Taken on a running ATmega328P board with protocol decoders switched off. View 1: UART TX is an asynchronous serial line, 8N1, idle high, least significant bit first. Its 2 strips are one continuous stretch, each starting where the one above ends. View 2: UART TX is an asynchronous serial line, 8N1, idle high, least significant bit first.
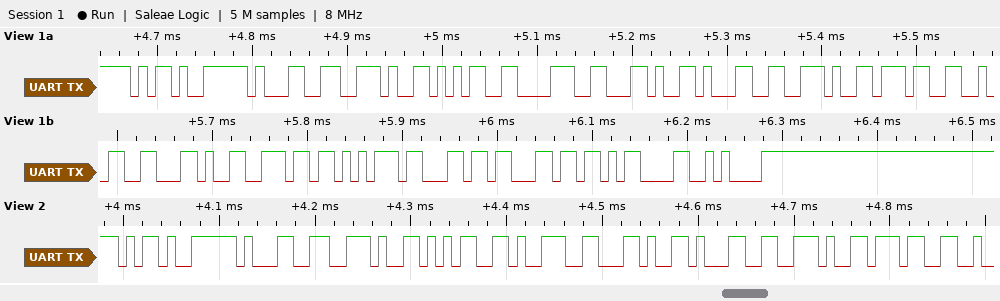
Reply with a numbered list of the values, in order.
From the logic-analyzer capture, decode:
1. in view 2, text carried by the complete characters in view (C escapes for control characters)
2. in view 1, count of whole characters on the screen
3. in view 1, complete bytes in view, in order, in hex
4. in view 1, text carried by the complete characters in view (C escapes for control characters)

1. "-1.59,1.7"
2. 17
3. 2D 31 2E 35 38 2C 31 2E 37 32 2C 6E 75 6C 6C 0D 0A
4. "-1.58,1.72,null\r\n"
